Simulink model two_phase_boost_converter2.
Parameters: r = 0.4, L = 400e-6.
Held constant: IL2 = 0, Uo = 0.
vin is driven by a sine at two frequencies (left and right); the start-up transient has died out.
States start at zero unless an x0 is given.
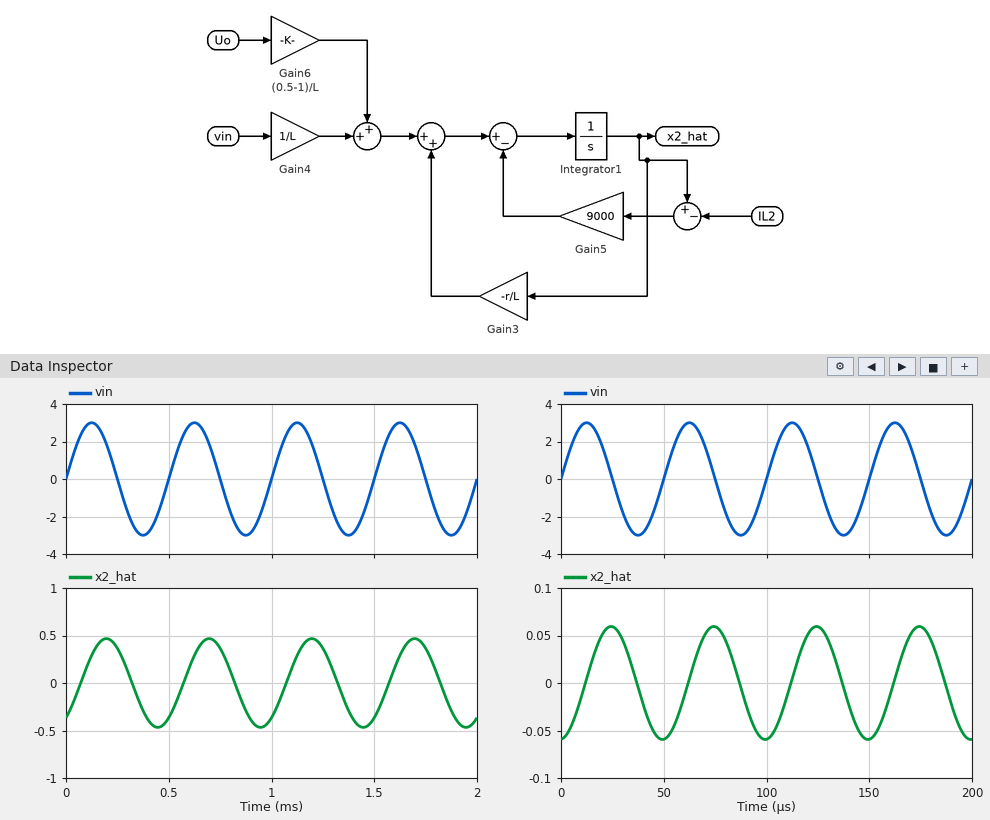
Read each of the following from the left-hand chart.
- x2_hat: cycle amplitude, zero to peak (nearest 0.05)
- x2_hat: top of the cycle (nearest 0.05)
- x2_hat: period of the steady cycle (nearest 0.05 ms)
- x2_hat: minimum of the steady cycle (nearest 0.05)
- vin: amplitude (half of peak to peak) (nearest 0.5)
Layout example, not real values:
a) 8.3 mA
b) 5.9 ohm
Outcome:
a) 0.45
b) 0.45
c) 0.50 ms
d) -0.45
e) 3.0
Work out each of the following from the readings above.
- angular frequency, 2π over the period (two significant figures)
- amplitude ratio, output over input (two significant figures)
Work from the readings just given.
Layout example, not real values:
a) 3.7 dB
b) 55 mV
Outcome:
a) 13 rad/ms
b) 0.15
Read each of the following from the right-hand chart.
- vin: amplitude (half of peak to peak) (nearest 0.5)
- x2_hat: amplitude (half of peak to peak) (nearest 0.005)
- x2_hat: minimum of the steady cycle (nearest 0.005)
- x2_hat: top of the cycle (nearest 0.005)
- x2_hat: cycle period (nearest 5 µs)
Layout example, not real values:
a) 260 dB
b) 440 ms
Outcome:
a) 3.0
b) 0.060
c) -0.060
d) 0.060
e) 50 µs
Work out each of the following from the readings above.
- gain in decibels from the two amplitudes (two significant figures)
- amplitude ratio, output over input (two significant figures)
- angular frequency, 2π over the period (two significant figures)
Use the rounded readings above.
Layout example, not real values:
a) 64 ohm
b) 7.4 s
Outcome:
a) -34 dB
b) 0.020
c) 0.13 rad/µs
